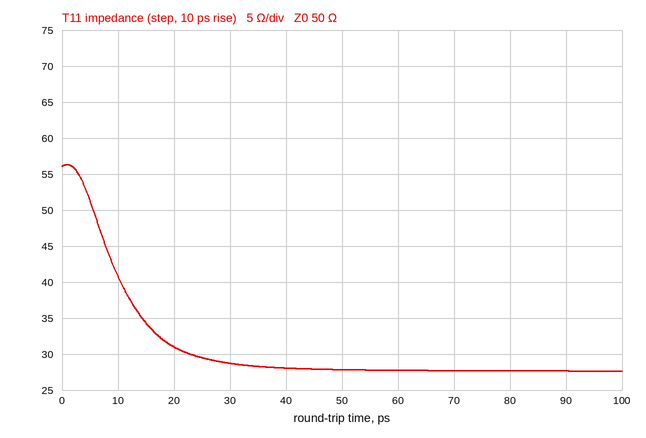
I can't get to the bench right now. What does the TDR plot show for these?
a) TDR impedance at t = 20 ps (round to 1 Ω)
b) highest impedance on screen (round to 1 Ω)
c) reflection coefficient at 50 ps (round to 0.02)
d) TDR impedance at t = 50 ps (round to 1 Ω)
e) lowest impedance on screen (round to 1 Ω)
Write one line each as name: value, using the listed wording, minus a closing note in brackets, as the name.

TDR impedance at t = 20 ps: 31 Ω
highest impedance on screen: 56 Ω
reflection coefficient at 50 ps: -0.28
TDR impedance at t = 50 ps: 28 Ω
lowest impedance on screen: 28 Ω
